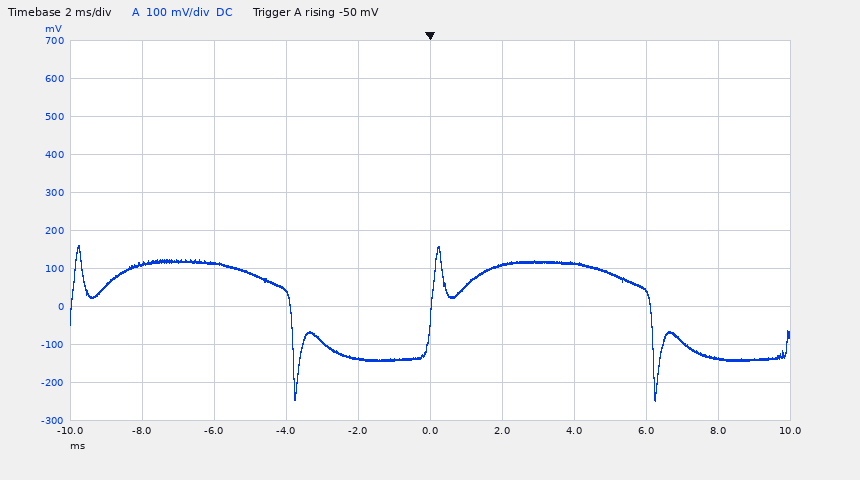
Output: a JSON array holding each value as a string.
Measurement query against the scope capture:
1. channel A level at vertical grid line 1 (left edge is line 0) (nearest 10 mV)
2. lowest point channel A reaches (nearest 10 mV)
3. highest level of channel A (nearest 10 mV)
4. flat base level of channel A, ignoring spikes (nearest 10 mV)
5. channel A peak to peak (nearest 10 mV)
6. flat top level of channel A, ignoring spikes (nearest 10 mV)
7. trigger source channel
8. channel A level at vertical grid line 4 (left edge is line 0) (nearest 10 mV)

["110 mV", "-250 mV", "160 mV", "-140 mV", "410 mV", "120 mV", "channel A", "-140 mV"]
